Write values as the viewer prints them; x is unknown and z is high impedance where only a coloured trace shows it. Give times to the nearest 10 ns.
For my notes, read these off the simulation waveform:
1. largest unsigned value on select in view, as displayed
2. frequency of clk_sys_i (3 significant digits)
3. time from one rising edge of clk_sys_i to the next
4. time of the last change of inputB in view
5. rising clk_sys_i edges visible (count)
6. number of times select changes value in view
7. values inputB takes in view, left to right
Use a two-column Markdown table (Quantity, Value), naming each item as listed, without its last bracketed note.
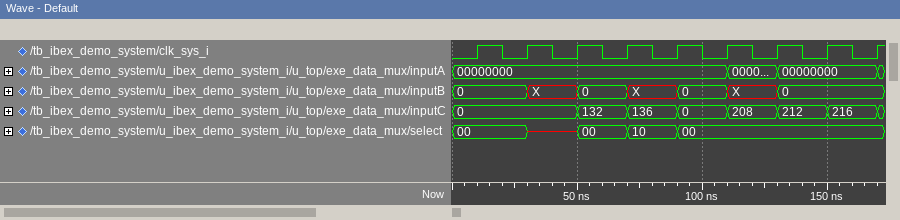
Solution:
| Quantity | Value |
|---|---|
| largest unsigned value on select in view, as displayed | 10 |
| frequency of clk_sys_i | 50.0 MHz |
| time from one rising edge of clk_sys_i to the next | 20 ns |
| time of the last change of inputB in view | 130 ns |
| rising clk_sys_i edges visible | 9 |
| number of times select changes value in view | 4 |
| values inputB takes in view, left to right | 0, X, 0, X, 0, X, 0 |
